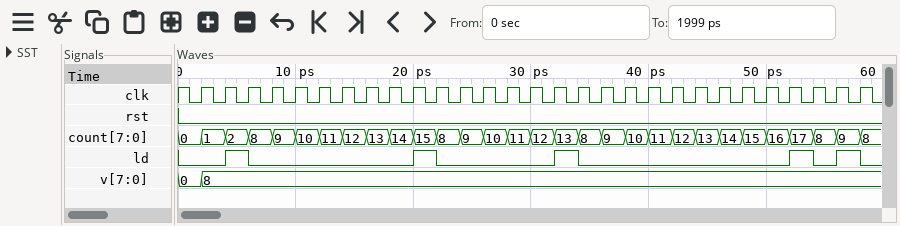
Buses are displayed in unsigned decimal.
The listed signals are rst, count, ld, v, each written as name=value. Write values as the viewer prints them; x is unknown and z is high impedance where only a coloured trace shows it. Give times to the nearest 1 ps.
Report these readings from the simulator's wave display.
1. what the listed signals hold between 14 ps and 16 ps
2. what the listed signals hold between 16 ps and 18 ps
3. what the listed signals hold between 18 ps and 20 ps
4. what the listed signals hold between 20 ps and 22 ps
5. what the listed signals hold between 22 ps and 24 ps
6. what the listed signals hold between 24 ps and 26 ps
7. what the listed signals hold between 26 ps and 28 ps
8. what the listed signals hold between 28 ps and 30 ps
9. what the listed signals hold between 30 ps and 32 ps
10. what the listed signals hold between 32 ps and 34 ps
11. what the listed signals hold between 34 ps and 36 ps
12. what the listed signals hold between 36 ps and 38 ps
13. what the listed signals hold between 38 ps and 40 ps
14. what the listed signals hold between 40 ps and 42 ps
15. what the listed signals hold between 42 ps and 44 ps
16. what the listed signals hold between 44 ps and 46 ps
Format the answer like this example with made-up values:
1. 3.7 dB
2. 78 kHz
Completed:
1. rst=0, count=12, ld=0, v=8
2. rst=0, count=13, ld=0, v=8
3. rst=0, count=14, ld=0, v=8
4. rst=0, count=15, ld=1, v=8
5. rst=0, count=8, ld=0, v=8
6. rst=0, count=9, ld=0, v=8
7. rst=0, count=10, ld=0, v=8
8. rst=0, count=11, ld=0, v=8
9. rst=0, count=12, ld=0, v=8
10. rst=0, count=13, ld=1, v=8
11. rst=0, count=8, ld=0, v=8
12. rst=0, count=9, ld=0, v=8
13. rst=0, count=10, ld=0, v=8
14. rst=0, count=11, ld=0, v=8
15. rst=0, count=12, ld=0, v=8
16. rst=0, count=13, ld=0, v=8
